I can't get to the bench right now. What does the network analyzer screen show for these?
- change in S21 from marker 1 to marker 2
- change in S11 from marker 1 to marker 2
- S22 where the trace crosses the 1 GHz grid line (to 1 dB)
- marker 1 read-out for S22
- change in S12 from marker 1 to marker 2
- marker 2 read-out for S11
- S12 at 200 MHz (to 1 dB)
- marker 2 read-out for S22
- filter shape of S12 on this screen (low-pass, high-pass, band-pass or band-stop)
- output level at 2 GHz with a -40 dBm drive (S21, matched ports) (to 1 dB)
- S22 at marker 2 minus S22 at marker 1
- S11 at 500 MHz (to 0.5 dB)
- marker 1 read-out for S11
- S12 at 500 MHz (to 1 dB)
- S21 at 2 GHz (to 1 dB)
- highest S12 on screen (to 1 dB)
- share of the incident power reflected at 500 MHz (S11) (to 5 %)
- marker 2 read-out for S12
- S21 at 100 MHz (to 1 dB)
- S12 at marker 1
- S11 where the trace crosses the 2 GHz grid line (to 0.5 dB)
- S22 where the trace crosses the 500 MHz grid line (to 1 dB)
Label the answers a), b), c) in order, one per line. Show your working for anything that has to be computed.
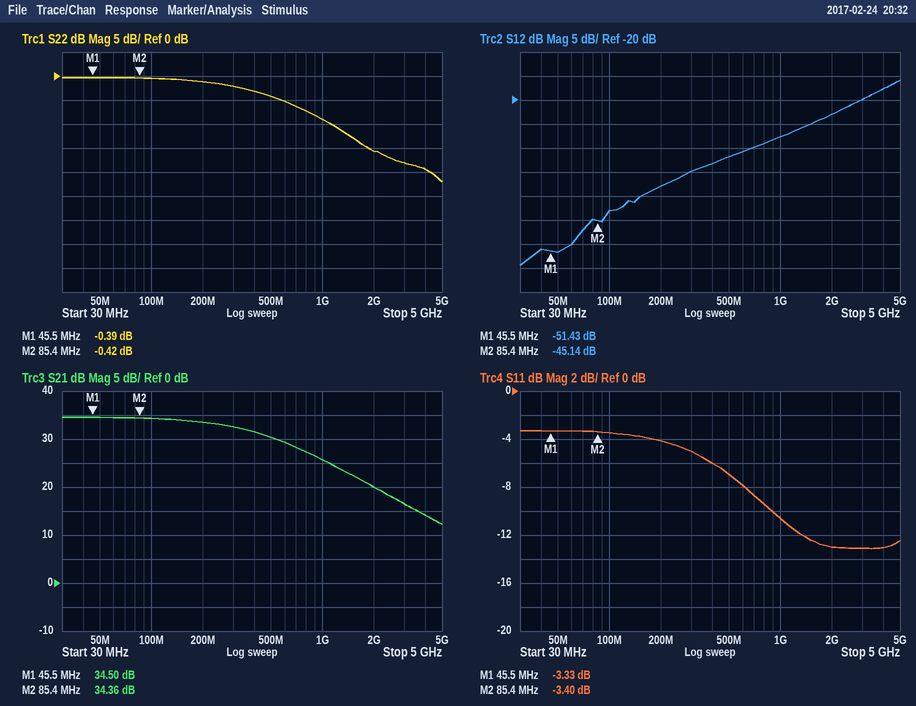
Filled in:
a) 34.36 − (34.5) = -0.14 dB
b) -3.4 − (-3.33) = -0.07 dB
c) -9 dB
d) -0.39 dB
e) -45.14 − (-51.43) = 6.29 dB
f) -3.40 dB
g) -38 dB
h) -0.42 dB
i) high-pass
j) -40 dBm + (20 dB) = -20 dBm
k) -0.42 − (-0.39) = -0.03 dB
l) -7.0 dB
m) -3.33 dB
n) -32 dB
o) 20 dB
p) -16 dB
q) 10^(-7/10) ≈ 20 %
r) -45.14 dB
s) 34 dB
t) -51.43 dB
u) -13.0 dB
v) -4 dB
